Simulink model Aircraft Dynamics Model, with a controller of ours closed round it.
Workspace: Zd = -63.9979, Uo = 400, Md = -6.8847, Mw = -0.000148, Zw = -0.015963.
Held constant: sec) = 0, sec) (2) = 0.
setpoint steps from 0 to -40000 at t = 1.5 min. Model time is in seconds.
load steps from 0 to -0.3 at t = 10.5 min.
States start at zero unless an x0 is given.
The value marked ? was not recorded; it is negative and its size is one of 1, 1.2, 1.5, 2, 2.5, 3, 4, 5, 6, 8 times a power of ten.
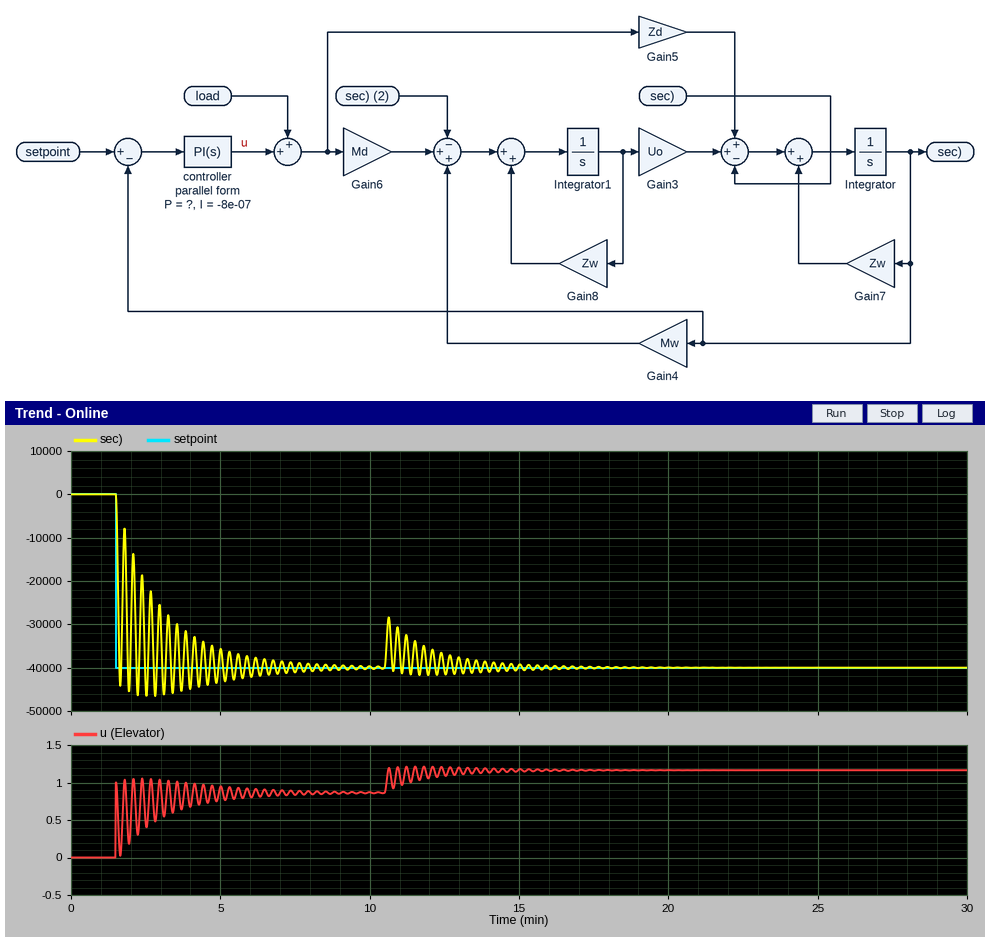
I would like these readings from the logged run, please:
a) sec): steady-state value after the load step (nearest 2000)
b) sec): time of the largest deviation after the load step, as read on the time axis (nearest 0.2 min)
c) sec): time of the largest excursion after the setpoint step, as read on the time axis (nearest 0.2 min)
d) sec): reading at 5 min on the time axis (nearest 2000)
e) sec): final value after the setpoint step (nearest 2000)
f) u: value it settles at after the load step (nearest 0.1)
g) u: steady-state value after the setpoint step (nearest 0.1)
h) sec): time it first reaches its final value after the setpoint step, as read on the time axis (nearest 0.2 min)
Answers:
-40000
10.6 min
2.8 min
-36000
-40000
1.2
0.9
1.6 min
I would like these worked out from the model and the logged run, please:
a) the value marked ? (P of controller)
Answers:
-2.5e-05
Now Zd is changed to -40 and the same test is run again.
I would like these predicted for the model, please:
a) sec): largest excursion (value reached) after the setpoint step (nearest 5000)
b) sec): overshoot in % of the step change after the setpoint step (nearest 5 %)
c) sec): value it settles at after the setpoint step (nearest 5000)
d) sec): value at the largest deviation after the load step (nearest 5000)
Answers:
-45000
15 %
-40000
-30000
